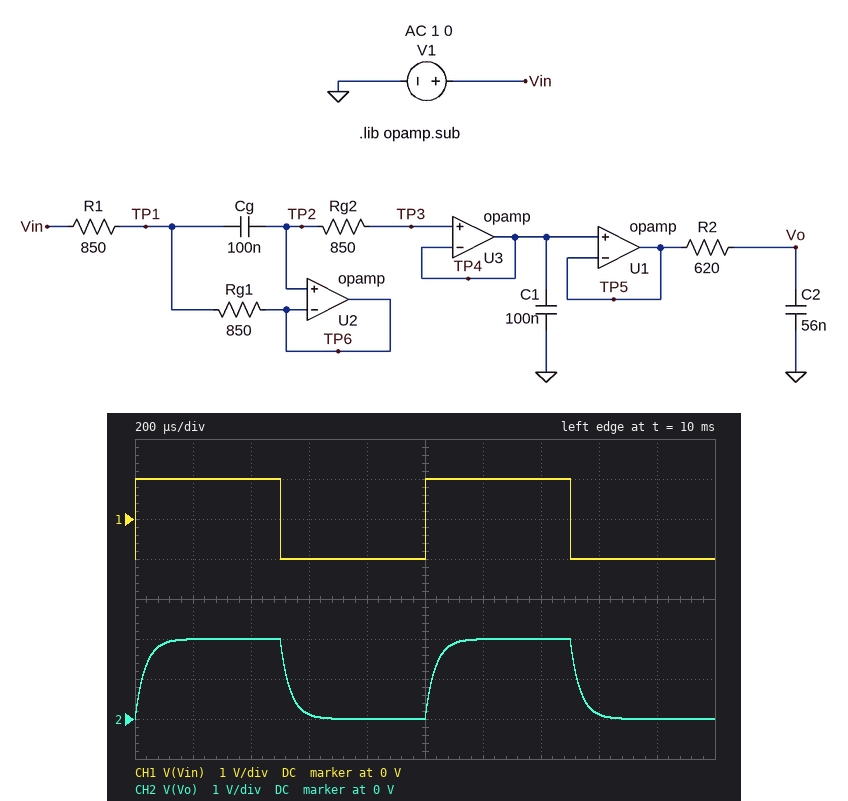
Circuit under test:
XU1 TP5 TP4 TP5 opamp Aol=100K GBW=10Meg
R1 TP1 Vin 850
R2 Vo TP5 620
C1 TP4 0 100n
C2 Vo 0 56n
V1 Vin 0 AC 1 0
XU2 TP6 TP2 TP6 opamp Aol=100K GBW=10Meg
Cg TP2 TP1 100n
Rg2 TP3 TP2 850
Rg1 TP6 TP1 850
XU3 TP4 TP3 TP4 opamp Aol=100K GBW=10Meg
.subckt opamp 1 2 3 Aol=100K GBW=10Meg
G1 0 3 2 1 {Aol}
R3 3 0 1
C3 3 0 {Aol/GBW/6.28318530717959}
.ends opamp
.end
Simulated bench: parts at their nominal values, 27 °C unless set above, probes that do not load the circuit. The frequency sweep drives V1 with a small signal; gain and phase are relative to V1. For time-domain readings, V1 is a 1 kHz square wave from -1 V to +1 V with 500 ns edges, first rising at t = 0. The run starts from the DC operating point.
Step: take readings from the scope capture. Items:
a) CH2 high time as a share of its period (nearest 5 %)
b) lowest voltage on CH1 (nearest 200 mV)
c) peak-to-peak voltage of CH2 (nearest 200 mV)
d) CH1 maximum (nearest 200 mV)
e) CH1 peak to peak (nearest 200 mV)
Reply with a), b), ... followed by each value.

a) 50 %
b) -1.0 V
c) 2.0 V
d) 1.0 V
e) 2.0 V
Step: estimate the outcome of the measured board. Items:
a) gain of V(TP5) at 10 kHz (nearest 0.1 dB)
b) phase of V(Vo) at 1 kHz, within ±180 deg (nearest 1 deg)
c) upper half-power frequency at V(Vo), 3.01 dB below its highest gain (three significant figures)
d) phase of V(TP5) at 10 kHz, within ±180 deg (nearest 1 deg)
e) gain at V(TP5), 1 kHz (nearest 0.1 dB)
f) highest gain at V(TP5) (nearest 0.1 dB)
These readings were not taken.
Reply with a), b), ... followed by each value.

a) 0 dB
b) -12 deg
c) 4.58 kHz
d) 0 deg
e) 0 dB
f) 0 dB
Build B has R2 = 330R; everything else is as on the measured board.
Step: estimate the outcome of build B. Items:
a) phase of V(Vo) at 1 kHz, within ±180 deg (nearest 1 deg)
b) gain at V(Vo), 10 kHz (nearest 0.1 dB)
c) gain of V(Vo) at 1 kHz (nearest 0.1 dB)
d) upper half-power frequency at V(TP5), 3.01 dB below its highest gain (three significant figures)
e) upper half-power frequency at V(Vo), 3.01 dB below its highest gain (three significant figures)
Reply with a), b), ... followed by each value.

a) -7 deg
b) -3.7 dB
c) -0.1 dB
d) 4.19 MHz
e) 8.61 kHz
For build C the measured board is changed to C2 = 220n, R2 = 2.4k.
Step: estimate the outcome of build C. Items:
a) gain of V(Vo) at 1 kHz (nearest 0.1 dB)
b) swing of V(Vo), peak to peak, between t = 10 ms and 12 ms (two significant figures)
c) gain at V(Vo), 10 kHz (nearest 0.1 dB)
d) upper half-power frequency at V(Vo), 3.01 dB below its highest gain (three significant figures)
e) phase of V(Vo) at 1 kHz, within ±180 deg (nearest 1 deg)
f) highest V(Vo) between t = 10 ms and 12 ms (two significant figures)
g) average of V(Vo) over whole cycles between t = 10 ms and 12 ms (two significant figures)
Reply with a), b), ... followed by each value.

a) -10.8 dB
b) 880 mV
c) -30.4 dB
d) 301 Hz
e) -73 deg
f) 1.4 V
g) 1.0 V
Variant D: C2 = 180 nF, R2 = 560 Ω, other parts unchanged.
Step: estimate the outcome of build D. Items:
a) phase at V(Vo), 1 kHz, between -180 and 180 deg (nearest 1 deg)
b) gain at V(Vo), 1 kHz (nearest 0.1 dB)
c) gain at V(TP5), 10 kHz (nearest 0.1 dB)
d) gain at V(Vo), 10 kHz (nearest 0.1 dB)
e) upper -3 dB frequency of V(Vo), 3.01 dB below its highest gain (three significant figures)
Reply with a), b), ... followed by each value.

a) -32 deg
b) -1.5 dB
c) 0 dB
d) -16.1 dB
e) 1.58 kHz
